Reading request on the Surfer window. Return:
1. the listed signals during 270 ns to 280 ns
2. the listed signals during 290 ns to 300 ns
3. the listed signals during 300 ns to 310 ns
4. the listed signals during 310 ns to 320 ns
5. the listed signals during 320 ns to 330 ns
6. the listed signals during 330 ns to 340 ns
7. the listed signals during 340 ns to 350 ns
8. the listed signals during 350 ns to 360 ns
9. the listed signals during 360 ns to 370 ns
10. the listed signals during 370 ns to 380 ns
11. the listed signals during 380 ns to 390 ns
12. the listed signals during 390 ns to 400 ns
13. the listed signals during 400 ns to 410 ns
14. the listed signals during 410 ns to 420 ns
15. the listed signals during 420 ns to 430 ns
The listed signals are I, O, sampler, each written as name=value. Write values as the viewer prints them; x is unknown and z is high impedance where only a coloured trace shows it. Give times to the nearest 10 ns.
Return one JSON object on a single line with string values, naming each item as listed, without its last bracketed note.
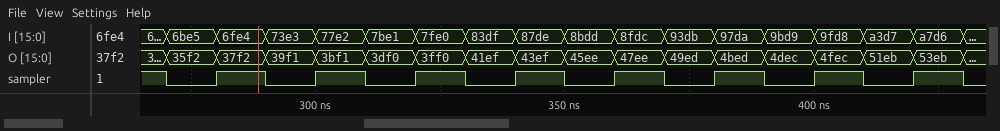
{"the listed signals during 270 ns to 280 ns": "I=6be5, O=35f2, sampler=0", "the listed signals during 290 ns to 300 ns": "I=73e3, O=39f1, sampler=0", "the listed signals during 300 ns to 310 ns": "I=77e2, O=3bf1, sampler=1", "the listed signals during 310 ns to 320 ns": "I=7be1, O=3df0, sampler=0", "the listed signals during 320 ns to 330 ns": "I=7fe0, O=3ff0, sampler=1", "the listed signals during 330 ns to 340 ns": "I=83df, O=41ef, sampler=0", "the listed signals during 340 ns to 350 ns": "I=87de, O=43ef, sampler=1", "the listed signals during 350 ns to 360 ns": "I=8bdd, O=45ee, sampler=0", "the listed signals during 360 ns to 370 ns": "I=8fdc, O=47ee, sampler=1", "the listed signals during 370 ns to 380 ns": "I=93db, O=49ed, sampler=0", "the listed signals during 380 ns to 390 ns": "I=97da, O=4bed, sampler=1", "the listed signals during 390 ns to 400 ns": "I=9bd9, O=4dec, sampler=0", "the listed signals during 400 ns to 410 ns": "I=9fd8, O=4fec, sampler=1", "the listed signals during 410 ns to 420 ns": "I=a3d7, O=51eb, sampler=0", "the listed signals during 420 ns to 430 ns": "I=a7d6, O=53eb, sampler=1"}
